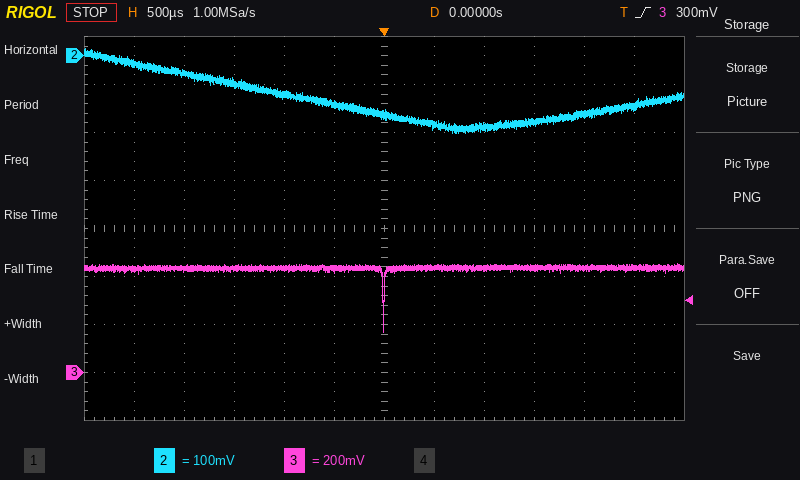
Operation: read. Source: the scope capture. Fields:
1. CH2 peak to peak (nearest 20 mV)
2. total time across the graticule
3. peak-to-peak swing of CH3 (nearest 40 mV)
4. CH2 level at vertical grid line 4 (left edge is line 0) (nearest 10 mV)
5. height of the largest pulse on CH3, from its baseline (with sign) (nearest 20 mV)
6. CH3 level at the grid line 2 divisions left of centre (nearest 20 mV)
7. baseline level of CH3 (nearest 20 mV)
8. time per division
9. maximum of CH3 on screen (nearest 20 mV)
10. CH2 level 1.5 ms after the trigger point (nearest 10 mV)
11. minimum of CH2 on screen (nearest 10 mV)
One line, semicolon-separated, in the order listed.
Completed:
180 mV; 6 ms; 280 mV; -80 mV; -260 mV; 440 mV; 440 mV; 500 µs; 460 mV; -140 mV; -160 mV
